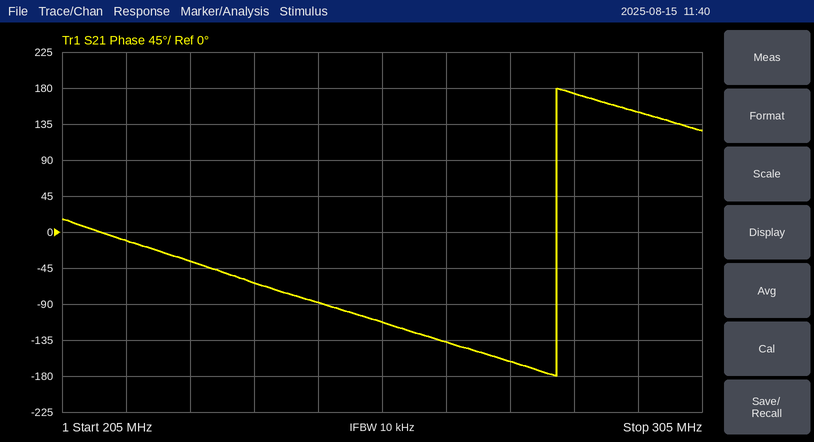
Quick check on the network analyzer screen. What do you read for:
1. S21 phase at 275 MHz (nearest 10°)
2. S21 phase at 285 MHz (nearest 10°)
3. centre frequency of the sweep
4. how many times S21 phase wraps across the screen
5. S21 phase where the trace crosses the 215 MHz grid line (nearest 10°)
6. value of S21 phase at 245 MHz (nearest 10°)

-160°
170°
255 MHz
1
-10°
-90°
